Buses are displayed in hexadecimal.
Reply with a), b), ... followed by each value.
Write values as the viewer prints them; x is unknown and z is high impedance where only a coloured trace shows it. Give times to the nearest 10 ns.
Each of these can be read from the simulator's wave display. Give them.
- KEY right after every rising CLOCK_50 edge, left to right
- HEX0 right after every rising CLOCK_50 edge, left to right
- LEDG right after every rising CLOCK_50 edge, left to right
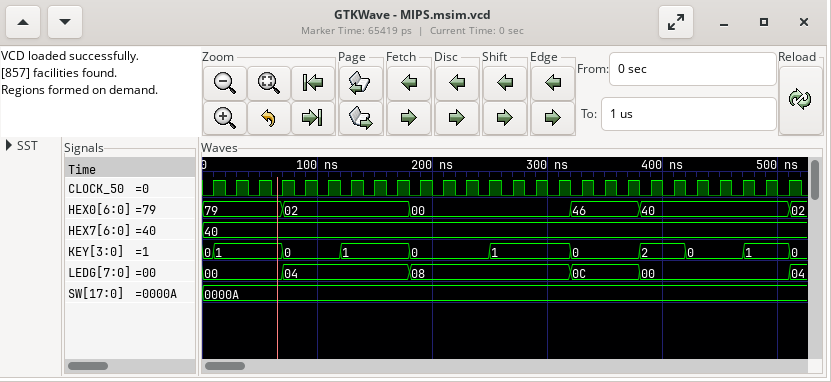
a) 1, 1, 1, 0, 0, 0, 1, 1, 1, 0, 0, 0, 1, 1, 1, 1, 0, 0, 0, 2, 2, 0, 0, 1, 1, 0
b) 79, 79, 79, 02, 02, 02, 02, 02, 02, 00, 00, 00, 00, 00, 00, 00, 46, 46, 46, 40, 40, 40, 40, 40, 40, 02
c) 00, 00, 00, 04, 04, 04, 04, 04, 04, 08, 08, 08, 08, 08, 08, 08, 0C, 0C, 0C, 00, 00, 00, 00, 00, 00, 04
